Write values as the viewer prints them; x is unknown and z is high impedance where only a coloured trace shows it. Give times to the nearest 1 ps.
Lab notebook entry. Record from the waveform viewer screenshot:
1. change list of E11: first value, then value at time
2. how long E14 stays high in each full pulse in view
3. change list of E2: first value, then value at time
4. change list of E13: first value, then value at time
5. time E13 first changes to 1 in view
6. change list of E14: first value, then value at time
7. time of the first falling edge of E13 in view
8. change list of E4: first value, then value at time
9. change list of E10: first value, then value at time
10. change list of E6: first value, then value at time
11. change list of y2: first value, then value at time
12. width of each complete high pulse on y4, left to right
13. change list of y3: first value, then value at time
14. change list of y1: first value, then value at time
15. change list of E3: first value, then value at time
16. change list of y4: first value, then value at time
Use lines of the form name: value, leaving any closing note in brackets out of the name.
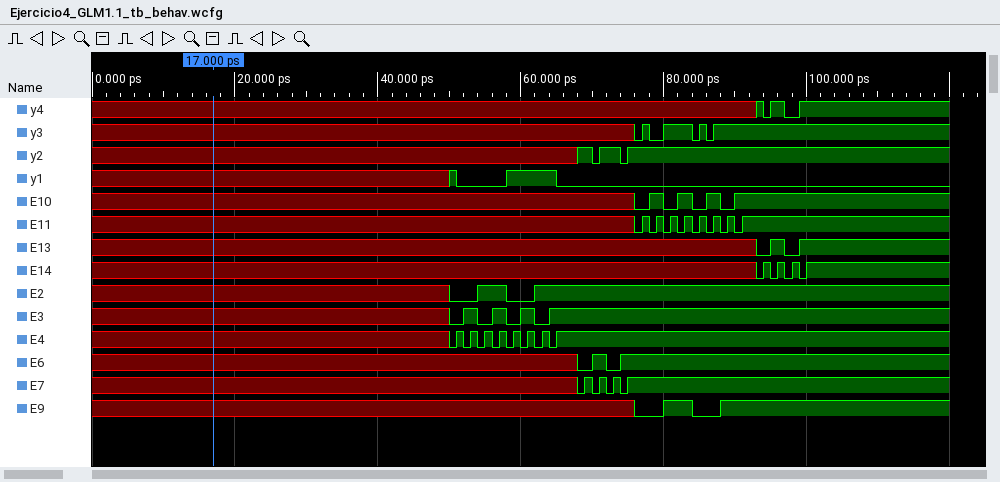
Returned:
change list of E11: first value, then value at time: x, 0 at 76 ps, 1 at 77 ps, 0 at 78 ps, 1 at 79 ps, 0 at 80 ps, 1 at 81 ps, 0 at 82 ps, 1 at 83 ps, 0 at 84 ps, 1 at 85 ps, 0 at 86 ps, 1 at 87 ps, 0 at 88 ps, 1 at 89 ps, 0 at 90 ps, 1 at 91 ps
how long E14 stays high in each full pulse in view: 1 ps, 1 ps, 1 ps
change list of E2: first value, then value at time: x, 0 at 50 ps, 1 at 54 ps, 0 at 58 ps, 1 at 62 ps
change list of E13: first value, then value at time: x, 0 at 93 ps, 1 at 95 ps, 0 at 97 ps, 1 at 99 ps
time E13 first changes to 1 in view: 95 ps
change list of E14: first value, then value at time: x, 0 at 93 ps, 1 at 94 ps, 0 at 95 ps, 1 at 96 ps, 0 at 97 ps, 1 at 98 ps, 0 at 99 ps, 1 at 100 ps
time of the first falling edge of E13 in view: 97 ps
change list of E4: first value, then value at time: x, 0 at 50 ps, 1 at 51 ps, 0 at 52 ps, 1 at 53 ps, 0 at 54 ps, 1 at 55 ps, 0 at 56 ps, 1 at 57 ps, 0 at 58 ps, 1 at 59 ps, 0 at 60 ps, 1 at 61 ps, 0 at 62 ps, 1 at 63 ps, 0 at 64 ps, 1 at 65 ps
change list of E10: first value, then value at time: x, 0 at 76 ps, 1 at 78 ps, 0 at 80 ps, 1 at 82 ps, 0 at 84 ps, 1 at 86 ps, 0 at 88 ps, 1 at 90 ps
change list of E6: first value, then value at time: x, 0 at 68 ps, 1 at 70 ps, 0 at 72 ps, 1 at 74 ps
change list of y2: first value, then value at time: x, 1 at 68 ps, 0 at 70 ps, 1 at 71 ps, 0 at 74 ps, 1 at 75 ps
width of each complete high pulse on y4, left to right: 2 ps
change list of y3: first value, then value at time: x, 0 at 76 ps, 1 at 77 ps, 0 at 78 ps, 1 at 80 ps, 0 at 84 ps, 1 at 85 ps, 0 at 86 ps, 1 at 87 ps
change list of y1: first value, then value at time: x, 1 at 50 ps, 0 at 51 ps, 1 at 58 ps, 0 at 65 ps
change list of E3: first value, then value at time: x, 0 at 50 ps, 1 at 52 ps, 0 at 54 ps, 1 at 56 ps, 0 at 58 ps, 1 at 60 ps, 0 at 62 ps, 1 at 64 ps
change list of y4: first value, then value at time: x, 1 at 93 ps, 0 at 94 ps, 1 at 95 ps, 0 at 97 ps, 1 at 99 ps
